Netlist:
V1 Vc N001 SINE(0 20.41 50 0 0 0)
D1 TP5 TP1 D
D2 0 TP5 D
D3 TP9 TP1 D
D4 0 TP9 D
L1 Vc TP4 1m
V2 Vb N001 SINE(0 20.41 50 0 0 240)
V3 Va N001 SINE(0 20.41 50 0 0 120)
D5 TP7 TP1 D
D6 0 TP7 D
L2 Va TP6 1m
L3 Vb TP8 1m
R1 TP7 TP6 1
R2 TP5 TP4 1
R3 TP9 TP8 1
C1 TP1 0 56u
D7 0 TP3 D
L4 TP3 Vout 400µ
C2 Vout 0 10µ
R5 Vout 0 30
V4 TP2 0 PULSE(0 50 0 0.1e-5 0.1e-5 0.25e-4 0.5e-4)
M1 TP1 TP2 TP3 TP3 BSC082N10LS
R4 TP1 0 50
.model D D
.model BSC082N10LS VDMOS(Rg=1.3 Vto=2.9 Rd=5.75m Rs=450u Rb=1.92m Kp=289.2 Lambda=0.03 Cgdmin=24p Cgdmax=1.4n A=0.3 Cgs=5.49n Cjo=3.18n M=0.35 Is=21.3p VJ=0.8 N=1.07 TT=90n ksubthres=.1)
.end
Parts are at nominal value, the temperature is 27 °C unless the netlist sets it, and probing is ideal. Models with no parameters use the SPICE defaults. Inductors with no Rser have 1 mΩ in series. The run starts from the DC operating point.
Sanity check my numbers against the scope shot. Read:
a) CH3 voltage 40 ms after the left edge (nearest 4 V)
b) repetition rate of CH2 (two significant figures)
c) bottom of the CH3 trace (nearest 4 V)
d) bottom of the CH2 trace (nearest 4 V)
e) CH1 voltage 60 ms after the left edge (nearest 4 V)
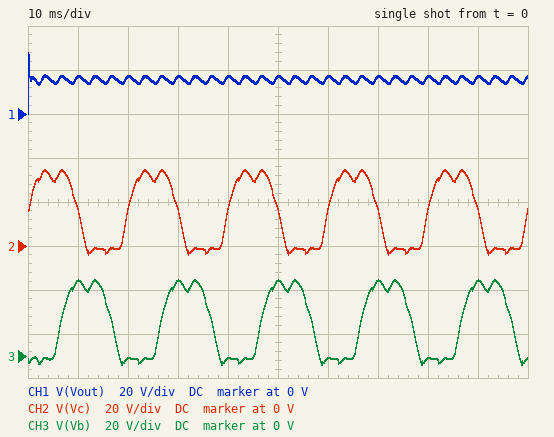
0 V
50 Hz
-4 V
-4 V
16 V
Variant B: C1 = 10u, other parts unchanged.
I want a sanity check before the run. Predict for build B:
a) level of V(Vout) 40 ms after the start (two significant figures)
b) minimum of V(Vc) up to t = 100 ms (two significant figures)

16 V
-4.1 V
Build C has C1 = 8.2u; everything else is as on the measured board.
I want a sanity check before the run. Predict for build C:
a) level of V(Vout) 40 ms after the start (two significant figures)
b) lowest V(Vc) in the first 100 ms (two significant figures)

16 V
-4.1 V
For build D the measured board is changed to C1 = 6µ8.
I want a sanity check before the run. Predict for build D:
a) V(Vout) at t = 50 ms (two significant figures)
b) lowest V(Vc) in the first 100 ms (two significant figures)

16 V
-4.1 V
